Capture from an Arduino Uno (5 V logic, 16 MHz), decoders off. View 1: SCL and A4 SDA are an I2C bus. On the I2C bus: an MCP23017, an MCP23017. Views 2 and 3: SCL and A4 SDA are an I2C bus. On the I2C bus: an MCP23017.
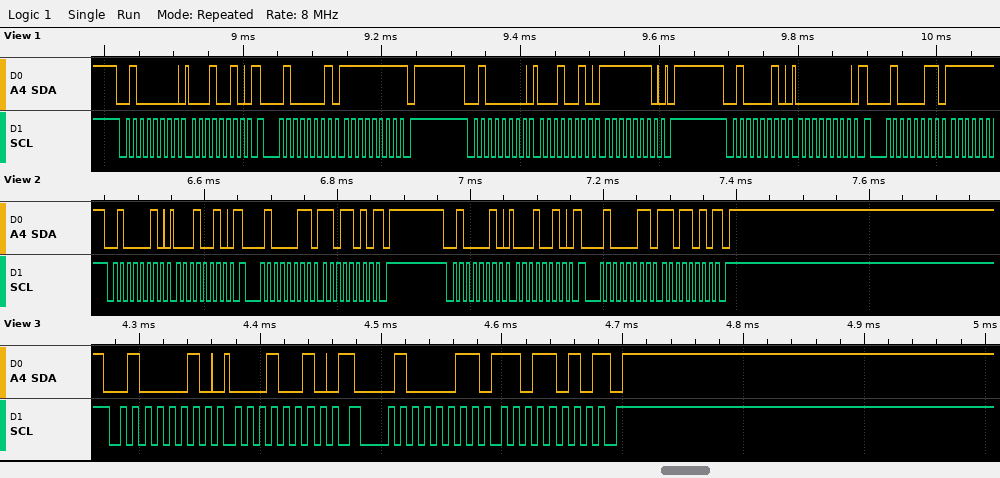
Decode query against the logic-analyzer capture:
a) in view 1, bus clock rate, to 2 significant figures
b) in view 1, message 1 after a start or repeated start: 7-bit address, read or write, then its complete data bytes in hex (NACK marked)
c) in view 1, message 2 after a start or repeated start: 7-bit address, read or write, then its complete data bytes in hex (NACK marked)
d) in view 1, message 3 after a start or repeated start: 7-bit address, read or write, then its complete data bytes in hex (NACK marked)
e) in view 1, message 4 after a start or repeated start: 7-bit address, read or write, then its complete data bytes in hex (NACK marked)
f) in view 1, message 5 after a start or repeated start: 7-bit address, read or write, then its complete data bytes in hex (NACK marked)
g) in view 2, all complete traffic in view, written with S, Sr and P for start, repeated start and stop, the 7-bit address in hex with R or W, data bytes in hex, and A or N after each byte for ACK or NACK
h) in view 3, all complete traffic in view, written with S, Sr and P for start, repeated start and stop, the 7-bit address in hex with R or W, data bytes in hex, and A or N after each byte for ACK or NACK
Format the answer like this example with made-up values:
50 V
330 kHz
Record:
100 kHz
0x20 write: 12
0x20 read: FF NACK
0x20 write: 12 FE
0x21 write: 00
0x21 read
S 21W A 12 A Sr 21R A DA N P S 21W A 12 A Sr 21R A DA N P
S 21W A 12 A Sr 21R A DA N P
